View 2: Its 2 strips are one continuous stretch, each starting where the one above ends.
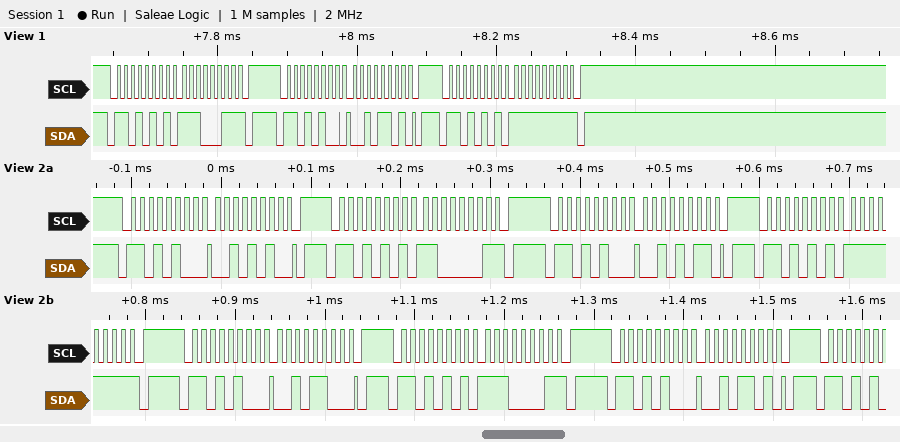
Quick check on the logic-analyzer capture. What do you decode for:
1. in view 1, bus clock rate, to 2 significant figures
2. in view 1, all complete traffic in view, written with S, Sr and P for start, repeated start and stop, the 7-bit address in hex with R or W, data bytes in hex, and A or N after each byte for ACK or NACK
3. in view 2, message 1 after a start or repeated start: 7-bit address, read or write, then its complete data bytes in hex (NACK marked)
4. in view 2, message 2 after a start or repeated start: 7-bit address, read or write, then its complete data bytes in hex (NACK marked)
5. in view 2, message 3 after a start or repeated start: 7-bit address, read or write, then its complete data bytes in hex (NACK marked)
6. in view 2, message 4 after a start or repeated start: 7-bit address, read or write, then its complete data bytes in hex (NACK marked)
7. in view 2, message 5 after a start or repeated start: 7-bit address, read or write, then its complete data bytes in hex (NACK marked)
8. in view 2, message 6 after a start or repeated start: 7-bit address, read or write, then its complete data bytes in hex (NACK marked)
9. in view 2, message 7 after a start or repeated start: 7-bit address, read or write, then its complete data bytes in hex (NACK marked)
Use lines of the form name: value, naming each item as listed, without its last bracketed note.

in view 1, bus clock rate, to 2 significant figures: 100 kHz
in view 1, all complete traffic in view, written with S, Sr and P for start, repeated start and stop, the 7-bit address in hex with R or W, data bytes in hex, and A or N after each byte for ACK or NACK: S 6AR A E3 N P S 6AW A 2D A P S 6AR A FF N P
in view 2, message 1 after a start or repeated start: 7-bit address, read or write, then its complete data bytes in hex: 0x6A write: 2A
in view 2, message 2 after a start or repeated start: 7-bit address, read or write, then its complete data bytes in hex: 0x6A read: C1 NACK
in view 2, message 3 after a start or repeated start: 7-bit address, read or write, then its complete data bytes in hex: 0x6A write: 2B
in view 2, message 4 after a start or repeated start: 7-bit address, read or write, then its complete data bytes in hex: 0x6A read: FF NACK
in view 2, message 5 after a start or repeated start: 7-bit address, read or write, then its complete data bytes in hex: 0x6A write: 2C
in view 2, message 6 after a start or repeated start: 7-bit address, read or write, then its complete data bytes in hex: 0x6A read: E1 NACK
in view 2, message 7 after a start or repeated start: 7-bit address, read or write, then its complete data bytes in hex: 0x6A write: 2D
